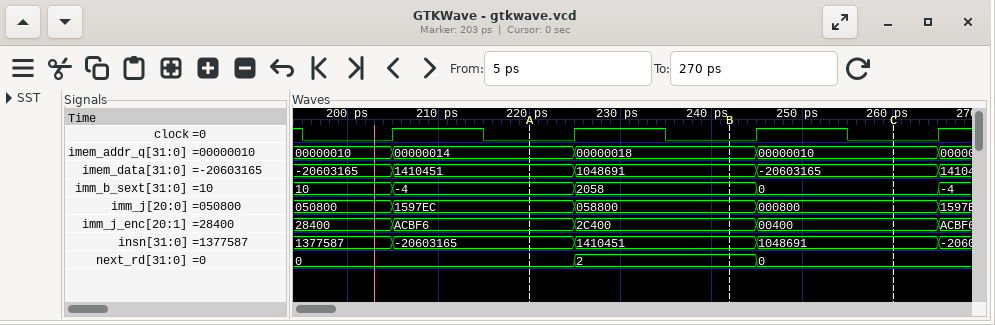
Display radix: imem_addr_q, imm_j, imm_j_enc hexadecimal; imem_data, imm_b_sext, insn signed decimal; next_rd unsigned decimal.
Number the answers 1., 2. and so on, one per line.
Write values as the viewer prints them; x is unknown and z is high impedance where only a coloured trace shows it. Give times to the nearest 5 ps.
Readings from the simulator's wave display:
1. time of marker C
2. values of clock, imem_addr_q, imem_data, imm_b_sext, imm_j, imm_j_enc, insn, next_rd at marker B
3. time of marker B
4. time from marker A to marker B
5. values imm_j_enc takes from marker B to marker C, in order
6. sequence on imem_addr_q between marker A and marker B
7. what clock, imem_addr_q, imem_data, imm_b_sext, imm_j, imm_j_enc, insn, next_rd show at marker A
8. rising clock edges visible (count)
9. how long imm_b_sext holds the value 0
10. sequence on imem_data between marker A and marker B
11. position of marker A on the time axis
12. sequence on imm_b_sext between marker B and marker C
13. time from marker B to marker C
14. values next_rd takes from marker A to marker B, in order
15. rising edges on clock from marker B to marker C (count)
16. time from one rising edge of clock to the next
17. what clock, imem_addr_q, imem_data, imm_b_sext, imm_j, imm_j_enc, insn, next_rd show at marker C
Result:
1. 260 ps
2. clock=0, imem_addr_q=00000018, imem_data=1048691, imm_b_sext=2058, imm_j=058800, imm_j_enc=2C400, insn=1410451, next_rd=2
3. 240 ps
4. 20 ps
5. 2C400, 00400
6. 00000014, 00000018
7. clock=0, imem_addr_q=00000014, imem_data=1410451, imm_b_sext=-4, imm_j=1597EC, imm_j_enc=ACBF6, insn=-20603165, next_rd=0
8. 4
9. 20 ps
10. 1410451, 1048691
11. 220 ps
12. 2058, 0
13. 20 ps
14. 0, 2
15. 1
16. 20 ps
17. clock=0, imem_addr_q=00000010, imem_data=-20603165, imm_b_sext=0, imm_j=000800, imm_j_enc=00400, insn=1048691, next_rd=0
